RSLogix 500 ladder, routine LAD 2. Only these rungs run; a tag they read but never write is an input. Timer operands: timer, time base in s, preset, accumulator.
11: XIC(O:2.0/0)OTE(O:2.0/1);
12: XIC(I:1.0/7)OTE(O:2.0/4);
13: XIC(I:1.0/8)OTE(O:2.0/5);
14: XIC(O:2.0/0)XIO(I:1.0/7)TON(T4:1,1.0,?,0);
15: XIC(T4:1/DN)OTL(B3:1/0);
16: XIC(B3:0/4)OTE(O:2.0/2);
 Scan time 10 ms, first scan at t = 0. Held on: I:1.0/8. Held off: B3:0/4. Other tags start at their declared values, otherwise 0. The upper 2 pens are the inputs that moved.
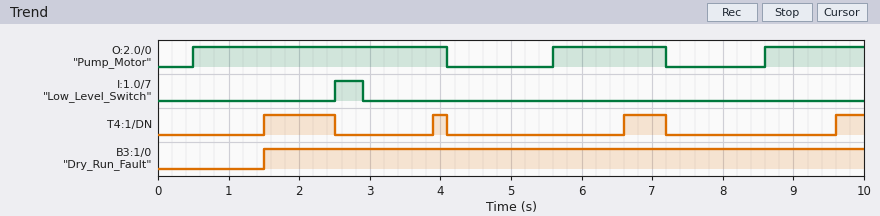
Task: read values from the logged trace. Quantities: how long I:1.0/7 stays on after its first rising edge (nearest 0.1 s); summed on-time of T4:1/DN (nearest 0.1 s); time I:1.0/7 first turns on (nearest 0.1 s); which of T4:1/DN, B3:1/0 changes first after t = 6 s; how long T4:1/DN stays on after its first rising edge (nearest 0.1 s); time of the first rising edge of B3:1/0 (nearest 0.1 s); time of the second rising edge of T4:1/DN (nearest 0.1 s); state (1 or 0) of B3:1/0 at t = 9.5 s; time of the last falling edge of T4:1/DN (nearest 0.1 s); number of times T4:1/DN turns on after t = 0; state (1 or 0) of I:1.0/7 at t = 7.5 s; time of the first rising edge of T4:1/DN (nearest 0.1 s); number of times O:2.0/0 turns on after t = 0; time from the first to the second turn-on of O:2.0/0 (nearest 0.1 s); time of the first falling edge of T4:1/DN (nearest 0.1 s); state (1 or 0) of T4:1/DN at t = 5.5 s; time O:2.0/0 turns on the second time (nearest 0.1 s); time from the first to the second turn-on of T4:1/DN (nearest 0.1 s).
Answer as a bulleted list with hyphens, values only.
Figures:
- 0.4 s
- 2.2 s
- 2.5 s
- T4:1/DN
- 1.0 s
- 1.5 s
- 3.9 s
- 1
- 7.2 s
- 4
- 0
- 1.5 s
- 3
- 5.1 s
- 2.5 s
- 0
- 5.6 s
- 2.4 s
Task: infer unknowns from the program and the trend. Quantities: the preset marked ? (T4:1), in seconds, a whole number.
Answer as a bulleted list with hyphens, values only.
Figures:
- 1 s
